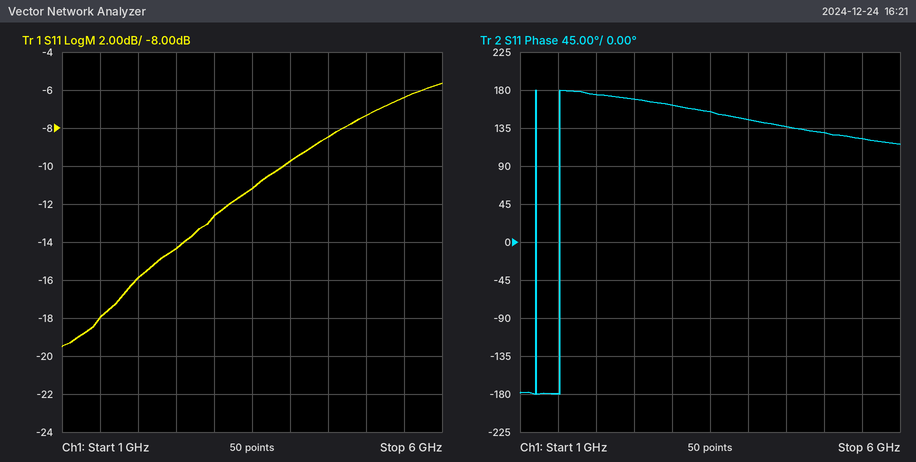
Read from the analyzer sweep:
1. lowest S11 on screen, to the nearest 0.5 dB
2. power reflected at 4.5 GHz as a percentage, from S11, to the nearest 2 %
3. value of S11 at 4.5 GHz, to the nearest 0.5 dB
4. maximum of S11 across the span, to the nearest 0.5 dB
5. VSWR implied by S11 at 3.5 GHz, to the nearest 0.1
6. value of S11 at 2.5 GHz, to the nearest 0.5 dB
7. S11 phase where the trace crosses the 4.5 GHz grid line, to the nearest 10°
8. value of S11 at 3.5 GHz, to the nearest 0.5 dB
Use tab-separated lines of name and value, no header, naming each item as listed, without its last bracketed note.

lowest S11 on screen, to the nearest 0.5 dB	-19.5 dB
power reflected at 4.5 GHz as a percentage, from S11, to the nearest 2 %	14 %
value of S11 at 4.5 GHz, to the nearest 0.5 dB	-8.5 dB
maximum of S11 across the span, to the nearest 0.5 dB	-5.5 dB
VSWR implied by S11 at 3.5 GHz, to the nearest 0.1	1.8
value of S11 at 2.5 GHz, to the nearest 0.5 dB	-14.5 dB
S11 phase where the trace crosses the 4.5 GHz grid line, to the nearest 10°	140°
value of S11 at 3.5 GHz, to the nearest 0.5 dB	-11.0 dB
